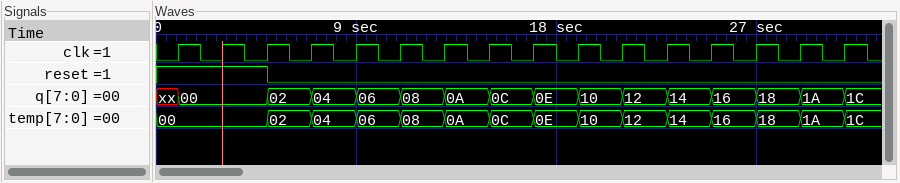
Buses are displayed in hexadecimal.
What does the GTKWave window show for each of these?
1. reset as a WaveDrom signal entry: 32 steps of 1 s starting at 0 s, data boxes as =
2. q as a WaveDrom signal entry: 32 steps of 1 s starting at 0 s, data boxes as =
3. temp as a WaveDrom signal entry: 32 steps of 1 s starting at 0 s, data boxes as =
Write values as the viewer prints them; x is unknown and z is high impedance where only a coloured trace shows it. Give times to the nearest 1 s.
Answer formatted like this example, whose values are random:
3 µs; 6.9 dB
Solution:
{name: 'reset', wave: '1....0..........................'}; {name: 'q', wave: 'x=...=.=.=.=.=.=.=.=.=.=.=.=.=.=', data: '00 02 04 06 08 0A 0C 0E 10 12 14 16 18 1A 1C'}; {name: 'temp', wave: '=....=.=.=.=.=.=.=.=.=.=.=.=.=.=', data: '00 02 04 06 08 0A 0C 0E 10 12 14 16 18 1A 1C'}
